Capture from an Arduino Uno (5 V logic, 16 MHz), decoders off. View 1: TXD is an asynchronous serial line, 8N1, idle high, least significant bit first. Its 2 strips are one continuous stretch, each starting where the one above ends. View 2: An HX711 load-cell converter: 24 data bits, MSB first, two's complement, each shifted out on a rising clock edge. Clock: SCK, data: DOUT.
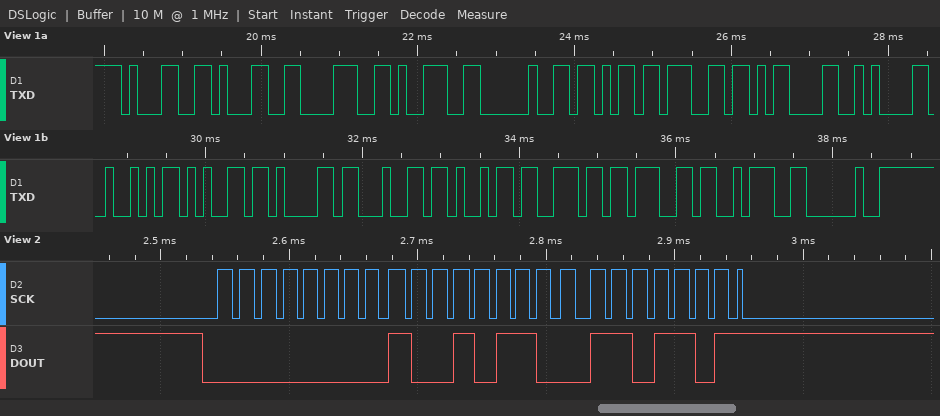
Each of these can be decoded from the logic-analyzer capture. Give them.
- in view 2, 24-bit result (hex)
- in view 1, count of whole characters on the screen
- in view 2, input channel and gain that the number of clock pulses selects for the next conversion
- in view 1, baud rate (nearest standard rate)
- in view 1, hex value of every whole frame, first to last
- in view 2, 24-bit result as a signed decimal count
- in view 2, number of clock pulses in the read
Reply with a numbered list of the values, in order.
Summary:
1. 0x00966D
2. 18
3. channel A, gain 128
4. 9600 baud
5. 0x31 0x31 0x38 0x39 0x20 0x6B 0x67 0x0D 0x0A 0x52 0x65 0x61 0x64 0x69 0x6E 0x67 0x3A 0x20
6. 38509
7. 25
